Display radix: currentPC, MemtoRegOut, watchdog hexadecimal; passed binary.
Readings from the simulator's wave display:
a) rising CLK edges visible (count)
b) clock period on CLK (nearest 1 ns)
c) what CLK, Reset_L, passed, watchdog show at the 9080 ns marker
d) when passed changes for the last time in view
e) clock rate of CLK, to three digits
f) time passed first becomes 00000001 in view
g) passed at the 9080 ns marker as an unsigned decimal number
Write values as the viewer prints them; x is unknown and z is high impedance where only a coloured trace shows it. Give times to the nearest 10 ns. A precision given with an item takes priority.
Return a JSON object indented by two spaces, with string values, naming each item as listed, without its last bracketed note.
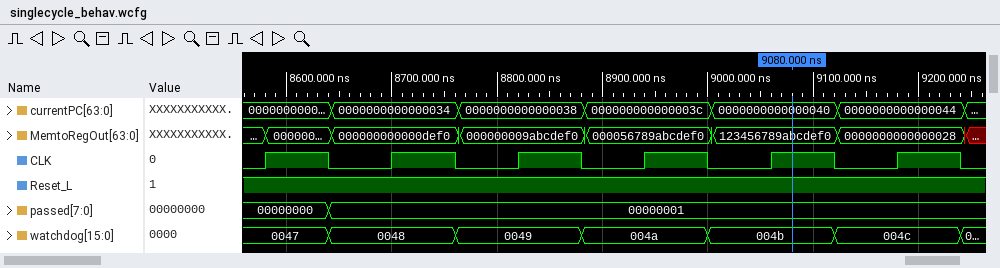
{
  "rising CLK edges visible": "6",
  "clock period on CLK": "120 ns",
  "what CLK, Reset_L, passed, watchdog show at the 9080 ns marker": "CLK=1, Reset_L=1, passed=00000001, watchdog=004b",
  "when passed changes for the last time in view": "8640 ns",
  "clock rate of CLK, to three digits": "8.33 MHz",
  "time passed first becomes 00000001 in view": "8640 ns",
  "passed at the 9080 ns marker as an unsigned decimal number": "1"
}
